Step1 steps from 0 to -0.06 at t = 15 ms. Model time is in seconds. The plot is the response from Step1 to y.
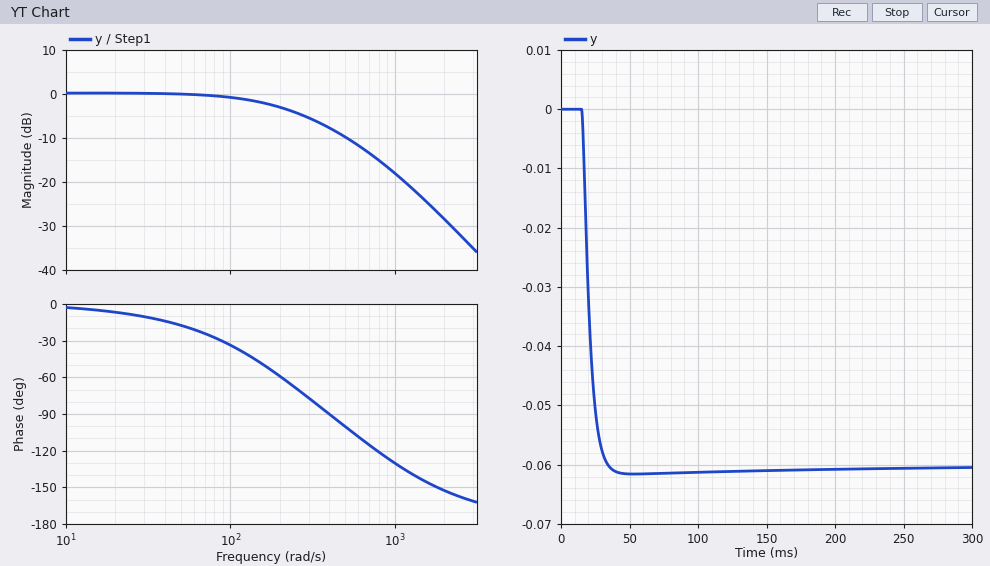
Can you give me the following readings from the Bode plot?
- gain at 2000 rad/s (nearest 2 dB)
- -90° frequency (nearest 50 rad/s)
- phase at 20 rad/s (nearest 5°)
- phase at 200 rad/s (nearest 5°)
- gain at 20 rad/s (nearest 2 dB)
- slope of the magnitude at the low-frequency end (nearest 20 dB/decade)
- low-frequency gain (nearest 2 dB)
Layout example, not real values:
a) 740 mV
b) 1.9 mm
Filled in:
a) -28 dB
b) 400 rad/s
c) -5°
d) -60°
e) 0 dB
f) 0 dB/decade
g) 0 dB
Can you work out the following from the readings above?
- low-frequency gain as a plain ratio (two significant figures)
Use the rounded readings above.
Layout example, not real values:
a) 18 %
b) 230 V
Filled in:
a) 1.0
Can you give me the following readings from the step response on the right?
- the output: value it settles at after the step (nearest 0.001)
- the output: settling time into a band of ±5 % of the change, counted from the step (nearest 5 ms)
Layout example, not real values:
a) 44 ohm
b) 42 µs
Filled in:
a) -0.060
b) 15 ms
